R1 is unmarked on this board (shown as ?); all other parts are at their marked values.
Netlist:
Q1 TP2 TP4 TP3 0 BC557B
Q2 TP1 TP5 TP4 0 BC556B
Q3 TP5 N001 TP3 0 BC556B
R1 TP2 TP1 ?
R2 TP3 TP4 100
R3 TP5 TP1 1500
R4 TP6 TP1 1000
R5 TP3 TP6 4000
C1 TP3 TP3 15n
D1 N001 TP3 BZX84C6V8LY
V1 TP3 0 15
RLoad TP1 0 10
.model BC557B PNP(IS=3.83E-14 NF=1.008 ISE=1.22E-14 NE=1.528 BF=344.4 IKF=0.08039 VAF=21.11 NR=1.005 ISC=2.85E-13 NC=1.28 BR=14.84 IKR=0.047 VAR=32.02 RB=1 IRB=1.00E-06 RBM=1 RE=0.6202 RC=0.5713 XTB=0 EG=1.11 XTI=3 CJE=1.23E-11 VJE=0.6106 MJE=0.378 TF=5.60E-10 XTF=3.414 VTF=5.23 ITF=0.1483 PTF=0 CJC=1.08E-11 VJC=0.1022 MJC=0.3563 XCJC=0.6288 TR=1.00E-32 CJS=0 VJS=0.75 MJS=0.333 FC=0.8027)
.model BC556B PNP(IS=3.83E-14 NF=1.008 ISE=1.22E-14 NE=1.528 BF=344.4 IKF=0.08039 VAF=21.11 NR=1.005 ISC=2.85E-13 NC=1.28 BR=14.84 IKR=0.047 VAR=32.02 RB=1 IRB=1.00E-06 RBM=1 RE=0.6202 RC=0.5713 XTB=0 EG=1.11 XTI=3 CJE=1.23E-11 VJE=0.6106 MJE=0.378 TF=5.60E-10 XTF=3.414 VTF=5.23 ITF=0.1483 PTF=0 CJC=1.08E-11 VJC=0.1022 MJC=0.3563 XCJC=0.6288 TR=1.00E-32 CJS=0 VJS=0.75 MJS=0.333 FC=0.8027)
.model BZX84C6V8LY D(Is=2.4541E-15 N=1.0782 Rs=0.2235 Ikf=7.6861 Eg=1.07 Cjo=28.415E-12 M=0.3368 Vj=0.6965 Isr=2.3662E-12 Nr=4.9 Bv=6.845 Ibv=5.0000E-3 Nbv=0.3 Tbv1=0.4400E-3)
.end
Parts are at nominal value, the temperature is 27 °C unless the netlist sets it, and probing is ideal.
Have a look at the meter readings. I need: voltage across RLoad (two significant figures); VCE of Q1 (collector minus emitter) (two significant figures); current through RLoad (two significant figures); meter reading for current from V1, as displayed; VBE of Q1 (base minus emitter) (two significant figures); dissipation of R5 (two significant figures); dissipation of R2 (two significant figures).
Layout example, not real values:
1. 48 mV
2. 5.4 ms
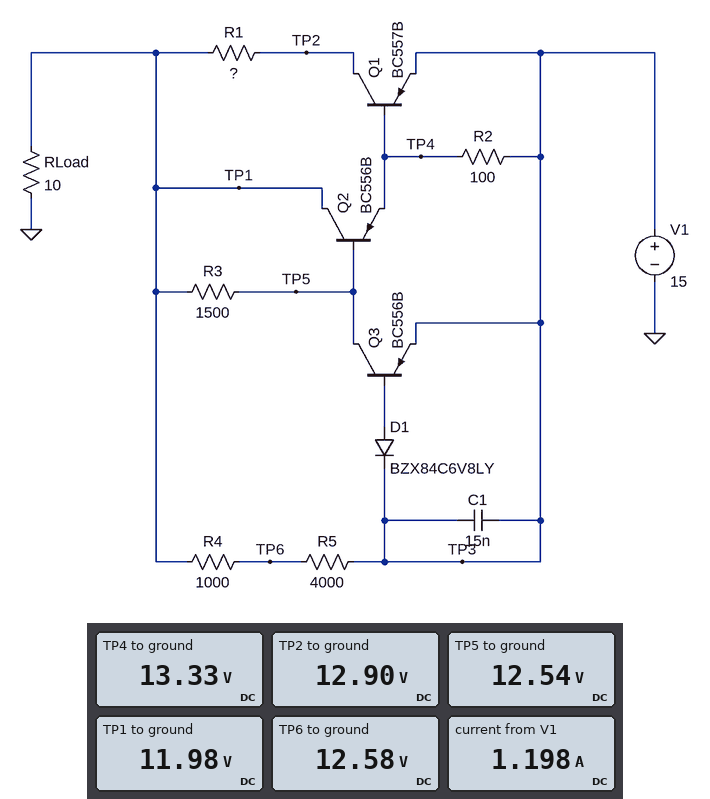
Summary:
1. 12 V
2. -2.1 V
3. 1.2 A
4. 1.198 A
5. -1.7 V
6. 1.5 mW
7. 28 mW
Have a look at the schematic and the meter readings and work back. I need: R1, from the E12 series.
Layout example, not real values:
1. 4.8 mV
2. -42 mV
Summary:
1. 0.82 Ω
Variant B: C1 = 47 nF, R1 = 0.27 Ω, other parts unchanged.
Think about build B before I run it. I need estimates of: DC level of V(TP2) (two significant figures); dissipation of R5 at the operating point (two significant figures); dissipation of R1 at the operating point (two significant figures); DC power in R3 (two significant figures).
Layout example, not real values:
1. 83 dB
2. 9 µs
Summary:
1. 12 V
2. 1.4 mW
3. 350 mW
4. 190 µW
